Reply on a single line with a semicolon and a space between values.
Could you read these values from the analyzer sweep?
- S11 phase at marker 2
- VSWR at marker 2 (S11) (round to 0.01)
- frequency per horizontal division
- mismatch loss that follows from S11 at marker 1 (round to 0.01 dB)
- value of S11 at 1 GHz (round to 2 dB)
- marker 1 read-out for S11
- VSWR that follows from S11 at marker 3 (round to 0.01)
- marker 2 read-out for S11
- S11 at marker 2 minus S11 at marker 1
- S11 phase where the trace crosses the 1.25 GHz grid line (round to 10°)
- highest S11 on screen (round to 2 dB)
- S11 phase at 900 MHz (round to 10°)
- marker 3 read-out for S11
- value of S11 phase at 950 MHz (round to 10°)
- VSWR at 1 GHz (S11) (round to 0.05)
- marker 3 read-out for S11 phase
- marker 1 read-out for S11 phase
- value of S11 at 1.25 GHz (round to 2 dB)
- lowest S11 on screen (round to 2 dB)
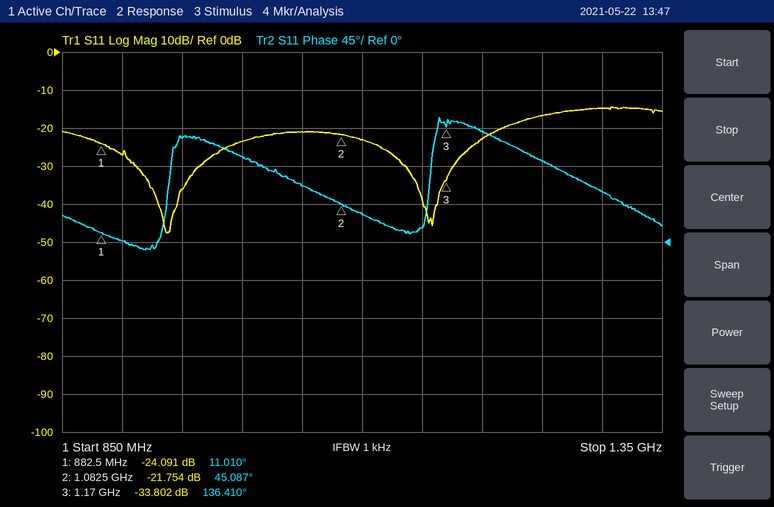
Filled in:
45.087°; 1.18; 50 MHz; 0.02 dB; -24 dB; -24.091 dB; 1.04; -21.754 dB; 2.337 dB; 100°; -14 dB; 0°; -33.802 dB; 120°; 1.15; 136.410°; 11.010°; -16 dB; -48 dB
